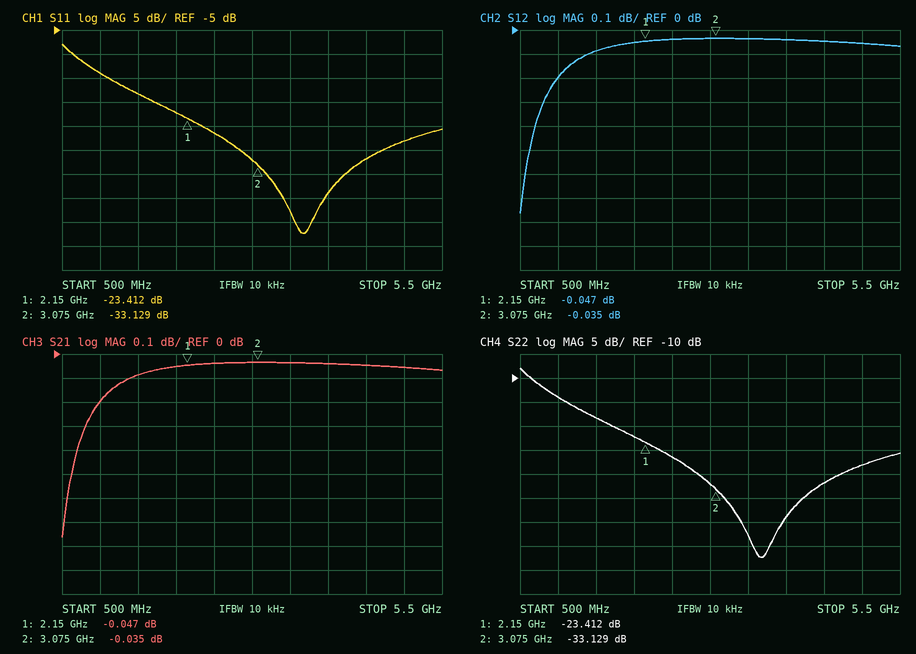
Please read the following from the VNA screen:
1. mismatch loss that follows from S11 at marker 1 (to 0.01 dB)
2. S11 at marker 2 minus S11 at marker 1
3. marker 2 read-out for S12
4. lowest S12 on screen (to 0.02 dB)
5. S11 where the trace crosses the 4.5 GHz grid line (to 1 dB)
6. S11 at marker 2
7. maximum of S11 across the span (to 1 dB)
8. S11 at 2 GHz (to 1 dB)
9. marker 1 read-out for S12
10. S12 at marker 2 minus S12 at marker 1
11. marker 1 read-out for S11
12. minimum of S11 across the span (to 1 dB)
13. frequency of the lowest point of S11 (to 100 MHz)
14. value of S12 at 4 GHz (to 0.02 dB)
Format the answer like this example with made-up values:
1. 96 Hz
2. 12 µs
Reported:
1. 0.02 dB
2. -9.717 dB
3. -0.035 dB
4. -0.76 dB
5. -32 dB
6. -33.129 dB
7. -8 dB
8. -22 dB
9. -0.047 dB
10. 0.012 dB
11. -23.412 dB
12. -47 dB
13. 3.7 GHz
14. -0.04 dB
